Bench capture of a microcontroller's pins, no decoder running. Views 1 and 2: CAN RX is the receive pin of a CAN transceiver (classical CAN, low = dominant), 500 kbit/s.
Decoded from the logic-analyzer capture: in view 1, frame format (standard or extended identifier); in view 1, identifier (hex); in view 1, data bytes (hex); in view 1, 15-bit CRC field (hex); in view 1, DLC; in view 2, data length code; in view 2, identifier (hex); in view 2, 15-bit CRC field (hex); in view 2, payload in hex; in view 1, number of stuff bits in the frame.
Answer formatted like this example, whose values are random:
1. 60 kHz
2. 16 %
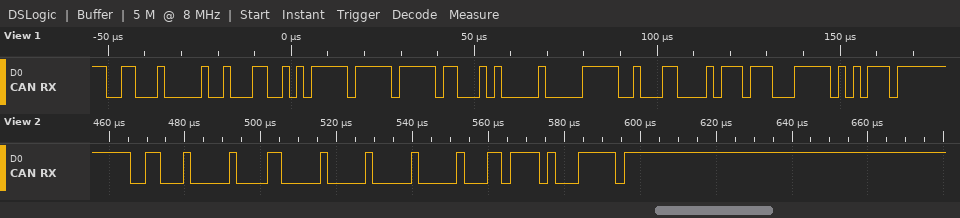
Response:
1. standard
2. 0x310
3. CA FF FF 8A 00 7A 30 BB
4. 0x47EB
5. 8
6. 3
7. 0x310
8. 0x5E8F
9. 00 00 01
10. 8
